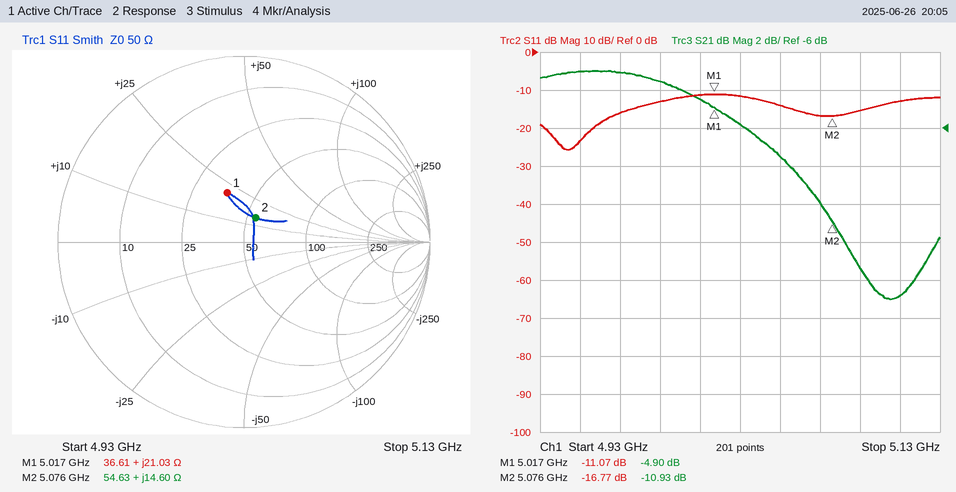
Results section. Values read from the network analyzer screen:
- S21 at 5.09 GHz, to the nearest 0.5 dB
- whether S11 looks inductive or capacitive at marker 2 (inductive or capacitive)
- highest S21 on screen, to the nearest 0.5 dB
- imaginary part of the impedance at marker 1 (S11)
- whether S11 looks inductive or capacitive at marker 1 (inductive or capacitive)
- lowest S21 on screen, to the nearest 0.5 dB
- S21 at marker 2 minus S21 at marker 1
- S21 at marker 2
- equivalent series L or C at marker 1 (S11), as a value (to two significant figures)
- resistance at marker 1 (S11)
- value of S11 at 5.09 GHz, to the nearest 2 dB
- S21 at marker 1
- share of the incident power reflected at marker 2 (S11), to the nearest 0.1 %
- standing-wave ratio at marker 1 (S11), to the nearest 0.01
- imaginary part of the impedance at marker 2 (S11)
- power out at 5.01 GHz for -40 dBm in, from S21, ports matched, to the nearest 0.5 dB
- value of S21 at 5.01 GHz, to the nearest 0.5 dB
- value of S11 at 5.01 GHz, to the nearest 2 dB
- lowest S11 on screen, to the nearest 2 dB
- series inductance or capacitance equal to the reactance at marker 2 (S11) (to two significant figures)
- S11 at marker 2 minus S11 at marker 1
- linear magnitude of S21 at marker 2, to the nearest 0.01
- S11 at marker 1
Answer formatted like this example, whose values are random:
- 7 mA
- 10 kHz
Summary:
- -13.5 dB
- inductive
- -3.0 dB
- +21.03 Ω
- inductive
- -15.0 dB
- -6.03 dB
- -10.93 dB
- 670 pH
- 36.61 Ω
- -16 dB
- -4.90 dB
- 2.1 %
- 1.78
- +14.60 Ω
- -44.5 dBm
- -4.5 dB
- -12 dB
- -26 dB
- 460 pH
- -5.70 dB
- 0.28
- -11.07 dB
